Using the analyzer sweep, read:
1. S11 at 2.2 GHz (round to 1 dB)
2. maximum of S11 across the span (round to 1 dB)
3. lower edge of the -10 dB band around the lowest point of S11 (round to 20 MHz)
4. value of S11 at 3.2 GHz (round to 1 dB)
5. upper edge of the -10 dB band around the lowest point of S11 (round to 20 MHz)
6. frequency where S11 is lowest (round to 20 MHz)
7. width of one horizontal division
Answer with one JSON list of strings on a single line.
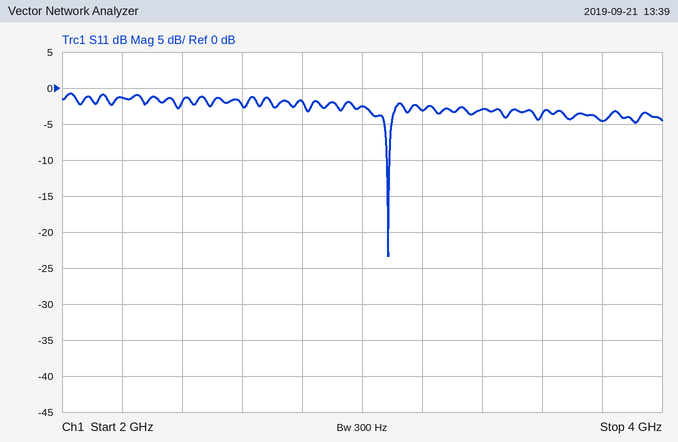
["-1 dB", "-1 dB", "3.08 GHz", "-3 dB", "3.10 GHz", "3.08 GHz", "200 MHz"]
